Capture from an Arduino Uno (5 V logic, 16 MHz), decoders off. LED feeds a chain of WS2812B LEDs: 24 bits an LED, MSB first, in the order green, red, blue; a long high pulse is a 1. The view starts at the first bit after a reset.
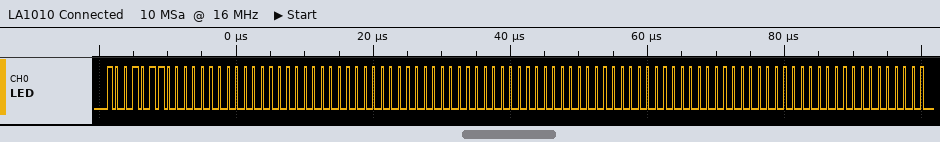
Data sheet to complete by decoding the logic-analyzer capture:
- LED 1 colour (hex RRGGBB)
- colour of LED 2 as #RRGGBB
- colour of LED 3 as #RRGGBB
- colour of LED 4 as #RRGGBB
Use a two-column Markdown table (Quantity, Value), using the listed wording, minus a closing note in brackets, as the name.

| Quantity | Value |
|---|---|
| LED 1 colour | #009600 |
| colour of LED 2 as #RRGGBB | #000000 |
| colour of LED 3 as #RRGGBB | #000000 |
| colour of LED 4 as #RRGGBB | #000000 |
